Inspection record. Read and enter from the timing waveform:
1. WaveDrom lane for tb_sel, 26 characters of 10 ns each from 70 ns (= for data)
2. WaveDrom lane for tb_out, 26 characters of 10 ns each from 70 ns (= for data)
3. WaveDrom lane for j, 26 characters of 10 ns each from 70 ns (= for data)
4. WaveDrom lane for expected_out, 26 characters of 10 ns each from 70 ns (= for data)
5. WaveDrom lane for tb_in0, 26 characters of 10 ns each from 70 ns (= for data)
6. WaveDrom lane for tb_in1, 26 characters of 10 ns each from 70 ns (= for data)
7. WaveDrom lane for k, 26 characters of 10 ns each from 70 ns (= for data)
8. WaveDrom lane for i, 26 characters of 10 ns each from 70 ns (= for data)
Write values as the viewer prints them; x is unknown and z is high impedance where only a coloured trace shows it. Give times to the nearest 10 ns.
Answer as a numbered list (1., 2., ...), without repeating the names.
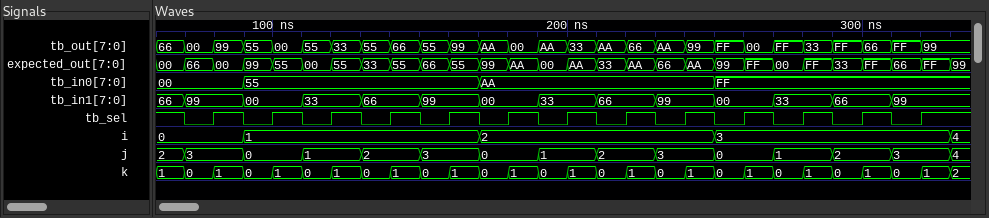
1. {name: 'tb_sel', wave: '01010101010101010101010101'}
2. {name: 'tb_out', wave: '==========================', data: '00 99 55 00 55 33 55 66 55 99 AA 00 AA 33 AA 66 AA 99 FF 00 FF 33 FF 66 FF 99'}
3. {name: 'j', wave: '=.=.=.=.=.=.=.=.=.=.=.=.=.', data: '3 0 1 2 3 0 1 2 3 0 1 2 3'}
4. {name: 'expected_out', wave: '==========================', data: '66 00 99 55 00 55 33 55 66 55 99 AA 00 AA 33 AA 66 AA 99 FF 00 FF 33 FF 66 FF'}
5. {name: 'tb_in0', wave: '=.=.......=.......=.......', data: '00 55 AA FF'}
6. {name: 'tb_in1', wave: '=.=.=.=.=.=.=.=.=.=.=.=.=.', data: '99 00 33 66 99 00 33 66 99 00 33 66 99'}
7. {name: 'k', wave: '==========================', data: '0 1 0 1 0 1 0 1 0 1 0 1 0 1 0 1 0 1 0 1 0 1 0 1 0 1'}
8. {name: 'i', wave: '=.=.......=.......=.......', data: '0 1 2 3'}
